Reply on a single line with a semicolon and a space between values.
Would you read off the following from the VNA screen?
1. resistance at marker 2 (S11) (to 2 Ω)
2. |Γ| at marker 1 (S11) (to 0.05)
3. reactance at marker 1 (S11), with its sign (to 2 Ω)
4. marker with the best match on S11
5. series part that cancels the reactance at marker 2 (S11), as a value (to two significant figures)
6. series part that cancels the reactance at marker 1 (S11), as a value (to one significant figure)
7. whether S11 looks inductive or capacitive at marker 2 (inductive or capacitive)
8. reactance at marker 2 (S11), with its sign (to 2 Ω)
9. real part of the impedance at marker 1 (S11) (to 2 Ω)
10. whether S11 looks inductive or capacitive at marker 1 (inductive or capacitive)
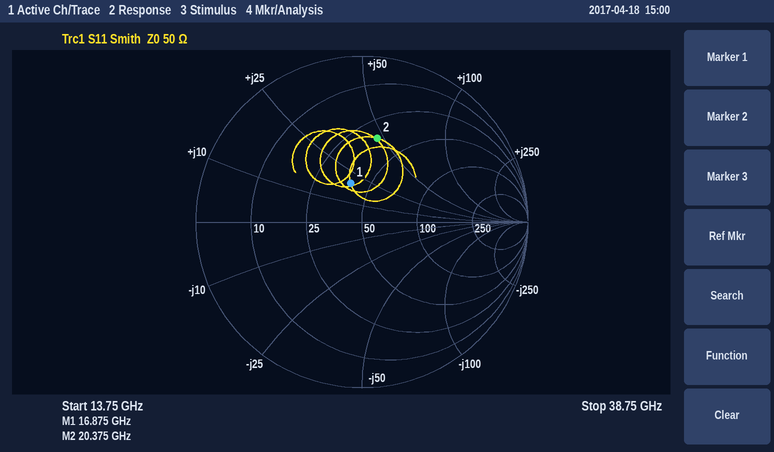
34 Ω; 0.25; +20 Ω; marker 1; 170 fF; 500 fF; inductive; +46 Ω; 40 Ω; inductive
